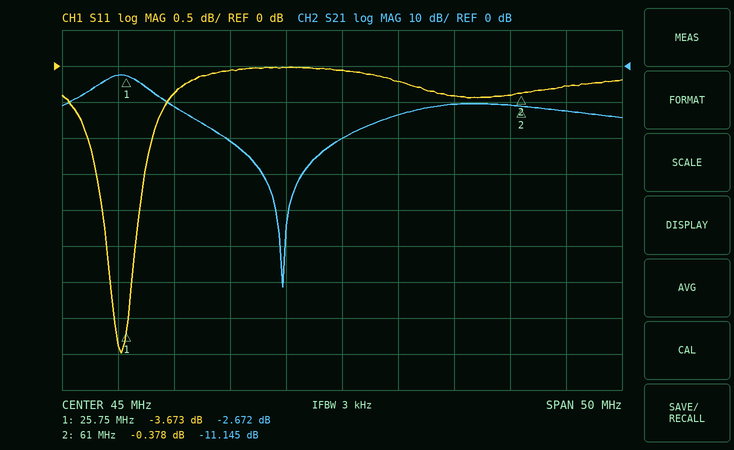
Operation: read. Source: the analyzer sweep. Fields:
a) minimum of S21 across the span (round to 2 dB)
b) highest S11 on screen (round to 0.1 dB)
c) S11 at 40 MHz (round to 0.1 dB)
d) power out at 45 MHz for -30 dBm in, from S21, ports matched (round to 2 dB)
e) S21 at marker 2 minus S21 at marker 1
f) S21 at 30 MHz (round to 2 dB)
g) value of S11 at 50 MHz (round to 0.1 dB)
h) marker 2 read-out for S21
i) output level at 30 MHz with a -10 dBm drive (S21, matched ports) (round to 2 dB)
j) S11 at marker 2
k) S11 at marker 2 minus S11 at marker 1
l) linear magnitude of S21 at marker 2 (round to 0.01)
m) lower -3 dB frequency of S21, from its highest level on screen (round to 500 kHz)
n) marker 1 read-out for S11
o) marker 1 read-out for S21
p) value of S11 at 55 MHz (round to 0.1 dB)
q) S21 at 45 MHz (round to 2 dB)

-62 dB
0.0 dB
0.0 dB
-50 dBm
-8.473 dB
-12 dB
-0.2 dB
-11.145 dB
-22 dBm
-0.378 dB
3.295 dB
0.28
23.0 MHz
-3.673 dB
-2.672 dB
-0.4 dB
-20 dB
